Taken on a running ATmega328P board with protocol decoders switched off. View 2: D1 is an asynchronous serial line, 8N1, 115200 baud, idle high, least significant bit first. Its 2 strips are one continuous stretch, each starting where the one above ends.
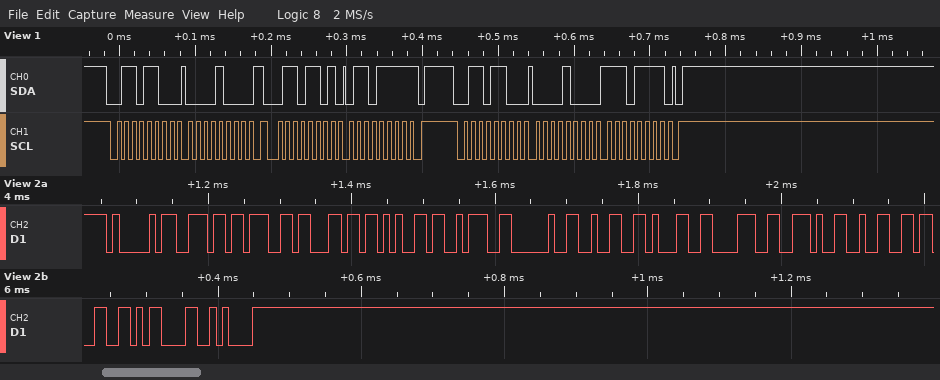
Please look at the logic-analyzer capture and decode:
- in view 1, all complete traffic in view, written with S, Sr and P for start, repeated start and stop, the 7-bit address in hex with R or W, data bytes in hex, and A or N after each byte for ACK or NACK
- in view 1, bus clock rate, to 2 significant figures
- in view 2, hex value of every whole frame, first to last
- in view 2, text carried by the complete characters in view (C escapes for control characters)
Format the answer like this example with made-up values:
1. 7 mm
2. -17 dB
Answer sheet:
1. S 36W A 08 A Sr 36R A 6F N P S 36W A 08 A EF A P
2. 100 kHz
3. 41 6E 67 6C 65 3A 20 32 31 38 2E 32 33 0D 0A
4. "Angle: 218.23\r\n"
